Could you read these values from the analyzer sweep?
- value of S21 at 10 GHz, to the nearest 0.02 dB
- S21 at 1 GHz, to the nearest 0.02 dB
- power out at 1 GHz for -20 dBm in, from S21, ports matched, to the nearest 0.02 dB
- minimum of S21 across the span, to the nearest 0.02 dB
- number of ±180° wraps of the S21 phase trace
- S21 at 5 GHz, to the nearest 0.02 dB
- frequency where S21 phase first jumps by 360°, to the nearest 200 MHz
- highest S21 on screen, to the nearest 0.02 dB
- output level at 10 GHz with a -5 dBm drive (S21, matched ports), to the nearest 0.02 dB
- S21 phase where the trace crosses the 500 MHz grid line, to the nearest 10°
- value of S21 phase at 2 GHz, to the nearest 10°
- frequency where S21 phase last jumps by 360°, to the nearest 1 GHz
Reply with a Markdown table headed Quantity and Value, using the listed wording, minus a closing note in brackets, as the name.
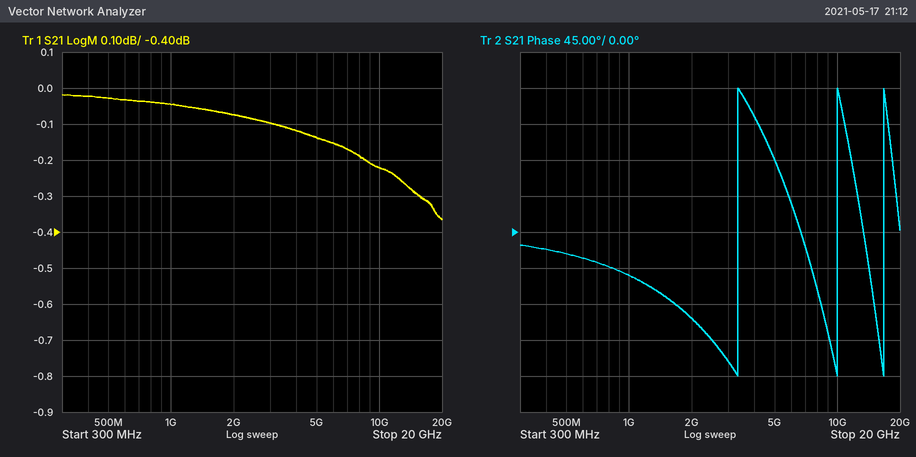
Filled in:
| Quantity | Value |
|---|---|
| value of S21 at 10 GHz, to the nearest 0.02 dB | -0.22 dB |
| S21 at 1 GHz, to the nearest 0.02 dB | -0.04 dB |
| power out at 1 GHz for -20 dBm in, from S21, ports matched, to the nearest 0.02 dB | -20.04 dBm |
| minimum of S21 across the span, to the nearest 0.02 dB | -0.36 dB |
| number of ±180° wraps of the S21 phase trace | 3 |
| S21 at 5 GHz, to the nearest 0.02 dB | -0.14 dB |
| frequency where S21 phase first jumps by 360°, to the nearest 200 MHz | 3.4 GHz |
| highest S21 on screen, to the nearest 0.02 dB | -0.02 dB |
| output level at 10 GHz with a -5 dBm drive (S21, matched ports), to the nearest 0.02 dB | -5.22 dBm |
| S21 phase where the trace crosses the 500 MHz grid line, to the nearest 10° | -30° |
| value of S21 phase at 2 GHz, to the nearest 10° | -110° |
| frequency where S21 phase last jumps by 360°, to the nearest 1 GHz | 17 GHz |
